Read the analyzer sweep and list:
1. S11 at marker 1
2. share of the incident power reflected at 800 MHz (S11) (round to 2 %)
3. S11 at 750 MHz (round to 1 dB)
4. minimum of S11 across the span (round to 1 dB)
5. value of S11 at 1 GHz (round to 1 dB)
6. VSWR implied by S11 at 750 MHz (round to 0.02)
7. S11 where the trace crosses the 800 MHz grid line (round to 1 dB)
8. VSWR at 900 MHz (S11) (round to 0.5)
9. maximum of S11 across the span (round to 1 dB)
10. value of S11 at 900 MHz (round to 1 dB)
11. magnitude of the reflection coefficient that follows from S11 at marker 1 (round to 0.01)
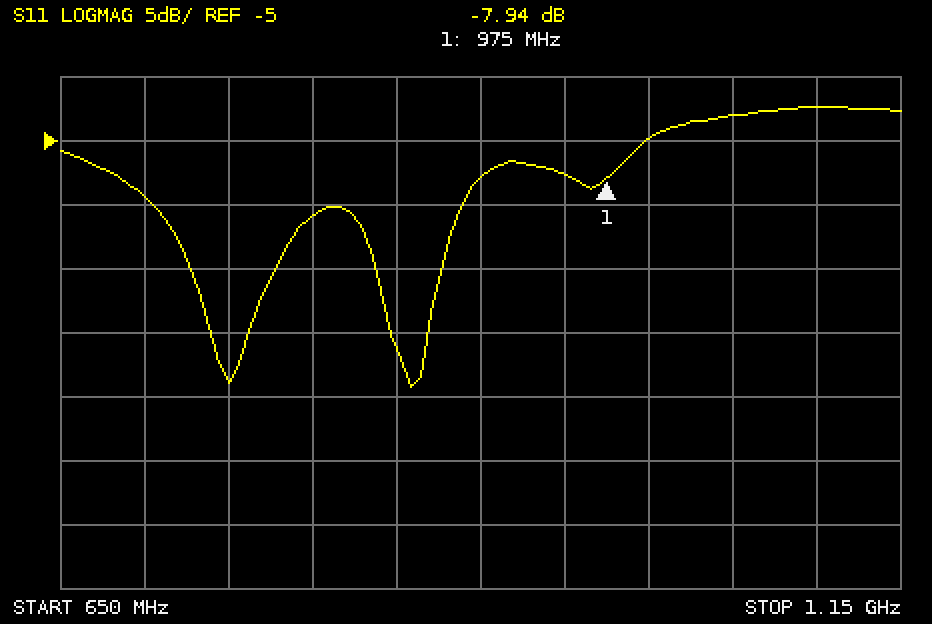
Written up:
-7.94 dB
8 %
-24 dB
-24 dB
-5 dB
1.14
-11 dB
2.5
-2 dB
-8 dB
0.40
